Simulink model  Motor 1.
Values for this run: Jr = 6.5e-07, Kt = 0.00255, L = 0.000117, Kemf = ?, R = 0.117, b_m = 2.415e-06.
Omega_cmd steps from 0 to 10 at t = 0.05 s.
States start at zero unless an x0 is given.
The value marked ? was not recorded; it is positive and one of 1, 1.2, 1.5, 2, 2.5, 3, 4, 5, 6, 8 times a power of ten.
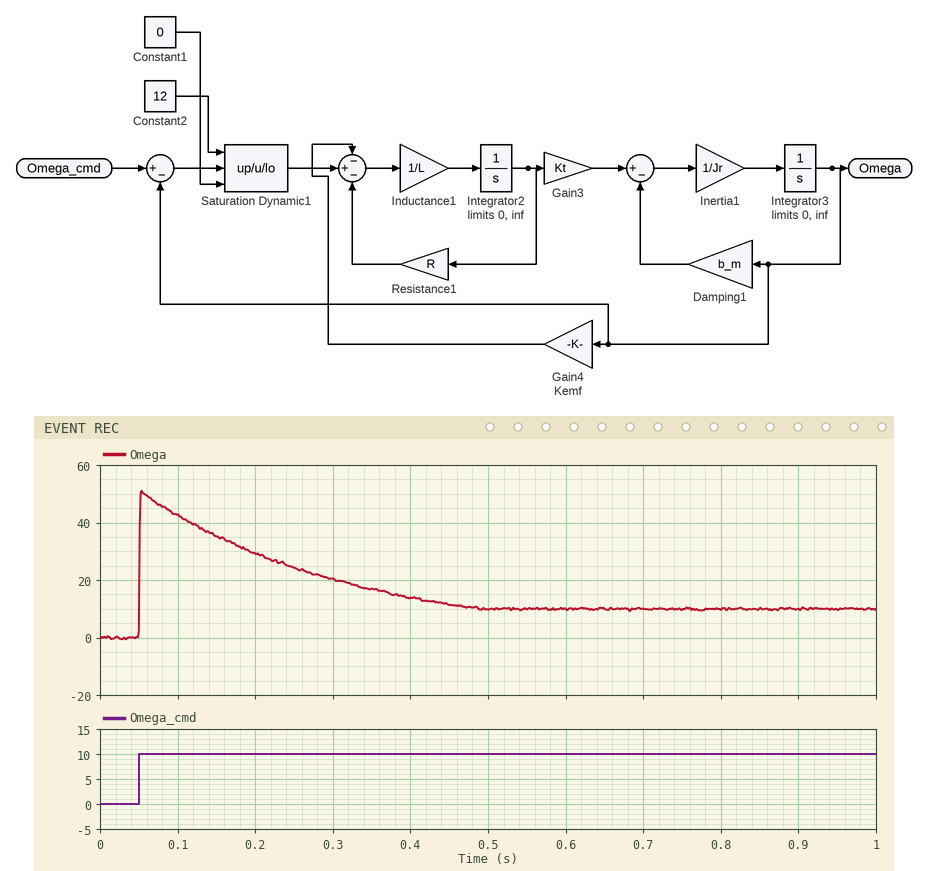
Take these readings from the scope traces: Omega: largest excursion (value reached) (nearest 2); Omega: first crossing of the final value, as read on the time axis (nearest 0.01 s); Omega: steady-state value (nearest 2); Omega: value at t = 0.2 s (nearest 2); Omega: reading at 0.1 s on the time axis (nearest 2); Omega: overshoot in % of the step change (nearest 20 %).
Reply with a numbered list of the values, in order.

1. 50
2. 0.05 s
3. 10
4. 30
5. 42
6. 400 %
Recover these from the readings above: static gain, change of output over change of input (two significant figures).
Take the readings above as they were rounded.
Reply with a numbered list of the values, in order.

1. 1.0
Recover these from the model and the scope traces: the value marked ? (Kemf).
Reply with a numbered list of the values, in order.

1. 0.0025
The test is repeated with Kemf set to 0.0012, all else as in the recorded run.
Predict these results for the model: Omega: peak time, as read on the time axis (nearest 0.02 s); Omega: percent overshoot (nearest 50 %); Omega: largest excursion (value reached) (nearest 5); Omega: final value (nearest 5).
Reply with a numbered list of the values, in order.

1. 0.06 s
2. 450 %
3. 55
4. 10
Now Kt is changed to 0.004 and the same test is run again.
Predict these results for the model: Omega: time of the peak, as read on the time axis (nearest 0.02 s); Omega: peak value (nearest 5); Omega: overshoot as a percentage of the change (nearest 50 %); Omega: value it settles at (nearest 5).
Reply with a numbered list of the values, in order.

1. 0.06 s
2. 60
3. 500 %
4. 10
